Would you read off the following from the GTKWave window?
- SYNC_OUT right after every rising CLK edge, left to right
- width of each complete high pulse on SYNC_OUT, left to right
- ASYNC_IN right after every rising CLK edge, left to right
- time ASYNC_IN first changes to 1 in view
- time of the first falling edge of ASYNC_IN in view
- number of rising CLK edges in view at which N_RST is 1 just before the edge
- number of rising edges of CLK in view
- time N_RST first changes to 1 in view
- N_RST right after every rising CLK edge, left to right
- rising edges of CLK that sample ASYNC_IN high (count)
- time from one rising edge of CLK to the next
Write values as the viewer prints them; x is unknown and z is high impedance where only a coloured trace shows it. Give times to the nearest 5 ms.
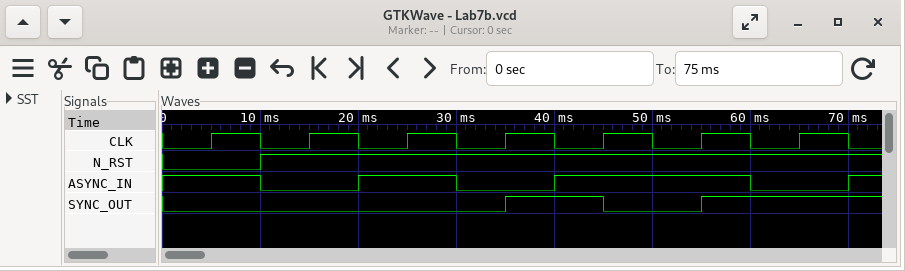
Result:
0 0 0 1 0 1 1
10 ms
1 0 1 0 1 1 0
20 ms
10 ms
6
7
10 ms
0 1 1 1 1 1 1
4
10 ms
